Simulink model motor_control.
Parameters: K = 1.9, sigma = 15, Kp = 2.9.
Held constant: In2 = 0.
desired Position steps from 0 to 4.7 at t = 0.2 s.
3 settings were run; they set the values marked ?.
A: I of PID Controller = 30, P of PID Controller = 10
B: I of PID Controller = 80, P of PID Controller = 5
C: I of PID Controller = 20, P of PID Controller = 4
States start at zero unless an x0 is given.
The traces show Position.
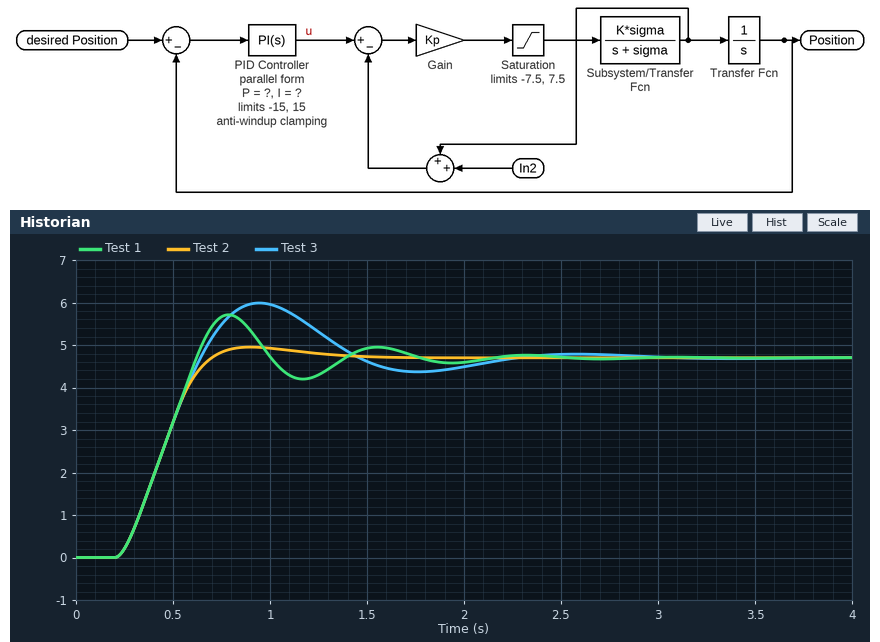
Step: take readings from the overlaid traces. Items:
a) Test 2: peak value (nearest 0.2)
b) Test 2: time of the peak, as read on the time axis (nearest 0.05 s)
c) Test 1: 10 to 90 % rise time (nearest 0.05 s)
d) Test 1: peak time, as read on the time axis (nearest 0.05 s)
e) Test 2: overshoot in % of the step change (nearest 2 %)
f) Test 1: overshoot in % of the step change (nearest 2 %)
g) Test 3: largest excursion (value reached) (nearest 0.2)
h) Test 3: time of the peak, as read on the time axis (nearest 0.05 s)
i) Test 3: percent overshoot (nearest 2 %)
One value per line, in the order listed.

5.0
0.90 s
0.30 s
0.80 s
6 %
22 %
6.0
0.95 s
28 %
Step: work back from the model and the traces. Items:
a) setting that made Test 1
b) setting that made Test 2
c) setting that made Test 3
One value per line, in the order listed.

B
A
C
